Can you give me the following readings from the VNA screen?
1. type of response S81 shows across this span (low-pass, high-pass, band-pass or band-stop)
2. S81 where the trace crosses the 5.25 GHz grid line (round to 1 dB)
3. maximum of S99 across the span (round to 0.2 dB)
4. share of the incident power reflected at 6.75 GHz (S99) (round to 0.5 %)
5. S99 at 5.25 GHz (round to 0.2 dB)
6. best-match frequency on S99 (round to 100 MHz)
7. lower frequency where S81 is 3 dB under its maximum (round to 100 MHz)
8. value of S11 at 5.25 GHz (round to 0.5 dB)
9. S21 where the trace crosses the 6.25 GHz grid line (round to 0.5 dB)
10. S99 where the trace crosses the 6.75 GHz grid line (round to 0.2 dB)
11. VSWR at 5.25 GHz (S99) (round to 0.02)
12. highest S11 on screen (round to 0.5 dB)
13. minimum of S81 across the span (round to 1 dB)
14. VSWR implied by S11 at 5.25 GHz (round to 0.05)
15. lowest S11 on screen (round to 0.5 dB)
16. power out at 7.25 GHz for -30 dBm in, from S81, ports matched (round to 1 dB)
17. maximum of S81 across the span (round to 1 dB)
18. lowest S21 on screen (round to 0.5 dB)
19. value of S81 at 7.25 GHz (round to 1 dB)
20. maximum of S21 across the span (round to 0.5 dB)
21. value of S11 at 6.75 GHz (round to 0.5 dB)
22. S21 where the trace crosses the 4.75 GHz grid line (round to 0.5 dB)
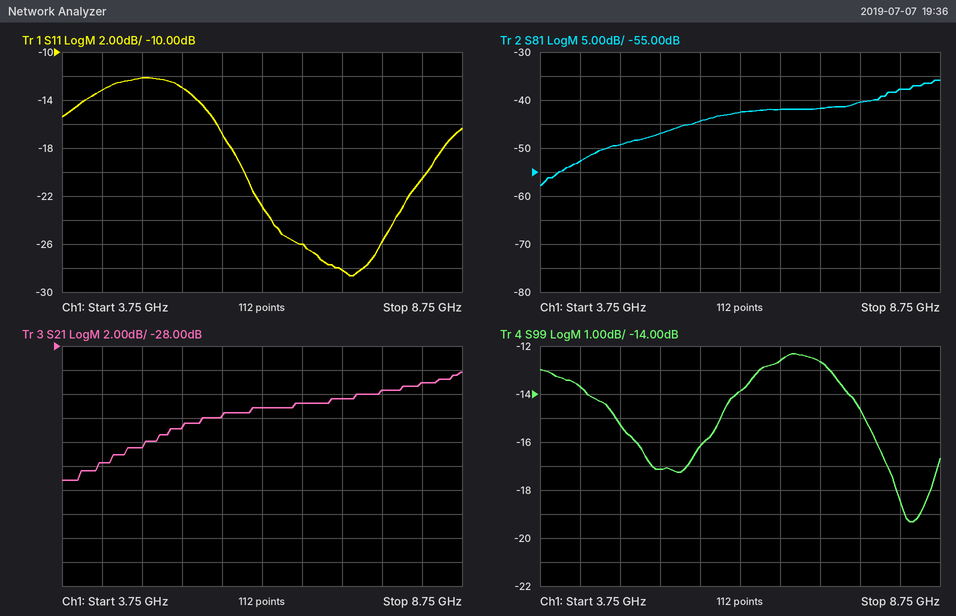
high-pass
-47 dB
-12.4 dB
5.5 %
-17.2 dB
8.4 GHz
8.1 GHz
-13.0 dB
-33.0 dB
-12.6 dB
1.32
-12.0 dB
-58 dB
1.60
-28.5 dB
-72 dBm
-36 dB
-39.0 dB
-42 dB
-30.0 dB
-26.0 dB
-36.5 dB
